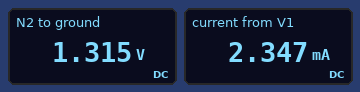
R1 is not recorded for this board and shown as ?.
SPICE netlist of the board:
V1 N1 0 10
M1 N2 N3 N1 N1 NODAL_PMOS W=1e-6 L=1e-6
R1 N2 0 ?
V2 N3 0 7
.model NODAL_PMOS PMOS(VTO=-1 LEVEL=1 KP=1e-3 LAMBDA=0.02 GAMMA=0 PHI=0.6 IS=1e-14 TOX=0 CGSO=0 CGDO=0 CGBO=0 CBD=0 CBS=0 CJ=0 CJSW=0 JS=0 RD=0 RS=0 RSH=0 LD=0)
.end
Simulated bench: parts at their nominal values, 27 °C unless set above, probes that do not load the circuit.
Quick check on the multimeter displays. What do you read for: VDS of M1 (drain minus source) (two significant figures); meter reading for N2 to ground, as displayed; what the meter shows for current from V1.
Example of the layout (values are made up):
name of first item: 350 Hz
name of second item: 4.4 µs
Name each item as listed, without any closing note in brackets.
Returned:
VDS of M1 (drain minus source): -8.7 V
meter reading for N2 to ground, as displayed: 1.315 V
what the meter shows for current from V1: 2.347 mA
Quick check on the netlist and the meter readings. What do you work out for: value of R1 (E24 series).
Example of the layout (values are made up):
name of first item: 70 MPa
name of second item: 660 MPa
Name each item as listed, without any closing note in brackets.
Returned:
value of R1: 560 Ω
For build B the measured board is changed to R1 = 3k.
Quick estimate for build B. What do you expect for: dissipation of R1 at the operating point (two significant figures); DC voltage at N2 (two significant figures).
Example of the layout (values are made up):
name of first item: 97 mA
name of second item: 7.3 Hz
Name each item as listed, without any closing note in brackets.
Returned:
dissipation of R1 at the operating point: 14 mW
DC voltage at N2: 6.4 V
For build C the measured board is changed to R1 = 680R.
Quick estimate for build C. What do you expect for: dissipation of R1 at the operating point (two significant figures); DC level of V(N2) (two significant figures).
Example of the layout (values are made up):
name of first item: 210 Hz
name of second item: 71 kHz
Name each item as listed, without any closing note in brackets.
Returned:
dissipation of R1 at the operating point: 3.7 mW
DC level of V(N2): 1.6 V
